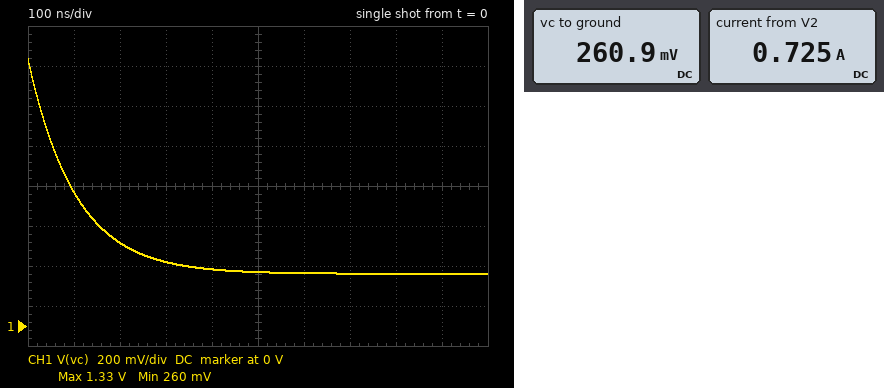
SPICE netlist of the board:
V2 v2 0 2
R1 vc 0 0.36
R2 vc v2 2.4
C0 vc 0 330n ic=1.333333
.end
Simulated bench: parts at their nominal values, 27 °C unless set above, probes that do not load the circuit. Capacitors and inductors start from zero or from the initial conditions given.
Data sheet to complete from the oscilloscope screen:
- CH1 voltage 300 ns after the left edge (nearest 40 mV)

320 mV
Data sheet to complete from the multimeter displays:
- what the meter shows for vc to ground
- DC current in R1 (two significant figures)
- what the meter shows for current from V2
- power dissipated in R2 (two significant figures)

260.9 mV
720 mA
0.725 A
1.3 W
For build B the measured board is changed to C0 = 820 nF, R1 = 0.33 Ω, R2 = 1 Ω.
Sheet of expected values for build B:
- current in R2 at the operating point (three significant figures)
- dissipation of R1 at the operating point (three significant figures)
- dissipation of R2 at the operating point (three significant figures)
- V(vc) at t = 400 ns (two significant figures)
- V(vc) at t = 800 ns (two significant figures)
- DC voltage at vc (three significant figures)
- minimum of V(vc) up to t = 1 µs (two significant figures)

1.50 A
746 mW
2.26 W
610 mV
510 mV
496 mV
500 mV
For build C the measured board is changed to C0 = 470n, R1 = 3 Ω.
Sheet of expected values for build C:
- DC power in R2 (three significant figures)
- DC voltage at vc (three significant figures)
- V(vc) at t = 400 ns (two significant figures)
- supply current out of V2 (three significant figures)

329 mW
1.11 V
1.2 V
370 mA
